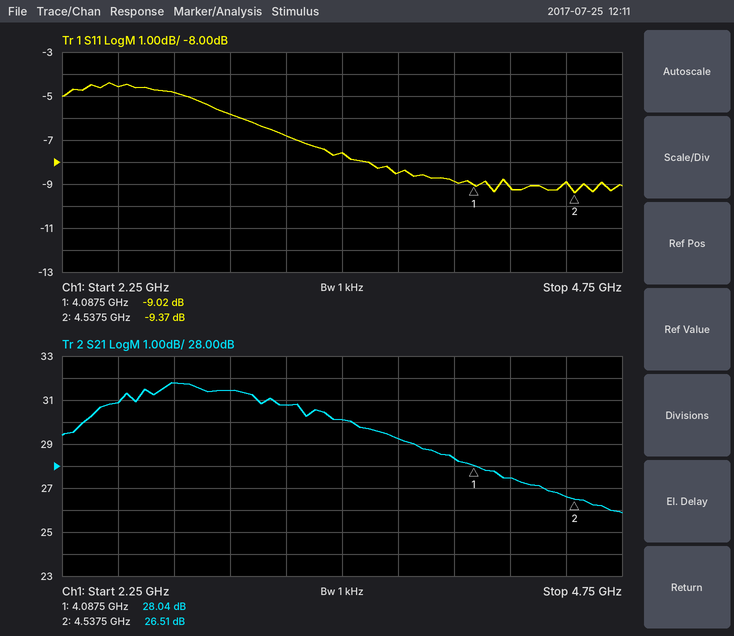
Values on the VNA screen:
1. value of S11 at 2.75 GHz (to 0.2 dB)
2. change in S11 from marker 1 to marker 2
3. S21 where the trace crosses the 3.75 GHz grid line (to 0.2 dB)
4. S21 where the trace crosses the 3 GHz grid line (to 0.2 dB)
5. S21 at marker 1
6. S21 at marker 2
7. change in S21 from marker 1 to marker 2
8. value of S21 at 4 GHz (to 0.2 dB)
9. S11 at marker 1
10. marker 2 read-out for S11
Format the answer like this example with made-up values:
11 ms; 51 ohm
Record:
-4.8 dB; -0.35 dB; 29.2 dB; 31.4 dB; 28.04 dB; 26.51 dB; -1.53 dB; 28.4 dB; -9.02 dB; -9.37 dB
